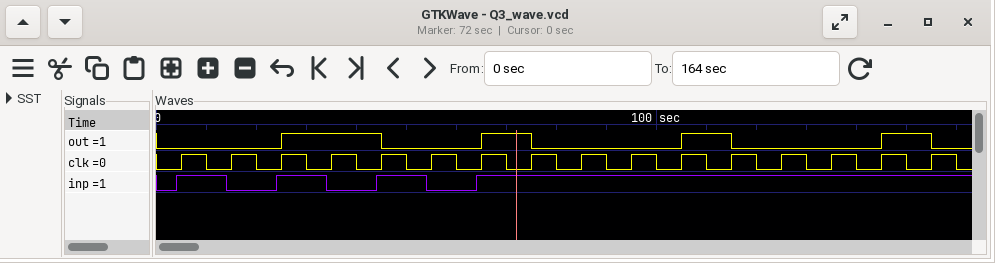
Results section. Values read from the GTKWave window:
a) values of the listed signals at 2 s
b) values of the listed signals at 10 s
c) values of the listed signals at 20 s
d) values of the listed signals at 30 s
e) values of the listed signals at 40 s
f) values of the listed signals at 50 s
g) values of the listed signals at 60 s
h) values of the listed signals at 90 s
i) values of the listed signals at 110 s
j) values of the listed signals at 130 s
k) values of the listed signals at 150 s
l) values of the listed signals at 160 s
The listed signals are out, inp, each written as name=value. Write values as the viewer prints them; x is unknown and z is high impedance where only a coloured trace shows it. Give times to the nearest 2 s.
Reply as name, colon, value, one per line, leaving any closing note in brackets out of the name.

values of the listed signals at 2 s: out=0, inp=0
values of the listed signals at 10 s: out=0, inp=1
values of the listed signals at 20 s: out=0, inp=0
values of the listed signals at 30 s: out=1, inp=1
values of the listed signals at 40 s: out=1, inp=0
values of the listed signals at 50 s: out=0, inp=1
values of the listed signals at 60 s: out=0, inp=0
values of the listed signals at 90 s: out=0, inp=1
values of the listed signals at 110 s: out=1, inp=1
values of the listed signals at 130 s: out=0, inp=1
values of the listed signals at 150 s: out=1, inp=1
values of the listed signals at 160 s: out=0, inp=1
